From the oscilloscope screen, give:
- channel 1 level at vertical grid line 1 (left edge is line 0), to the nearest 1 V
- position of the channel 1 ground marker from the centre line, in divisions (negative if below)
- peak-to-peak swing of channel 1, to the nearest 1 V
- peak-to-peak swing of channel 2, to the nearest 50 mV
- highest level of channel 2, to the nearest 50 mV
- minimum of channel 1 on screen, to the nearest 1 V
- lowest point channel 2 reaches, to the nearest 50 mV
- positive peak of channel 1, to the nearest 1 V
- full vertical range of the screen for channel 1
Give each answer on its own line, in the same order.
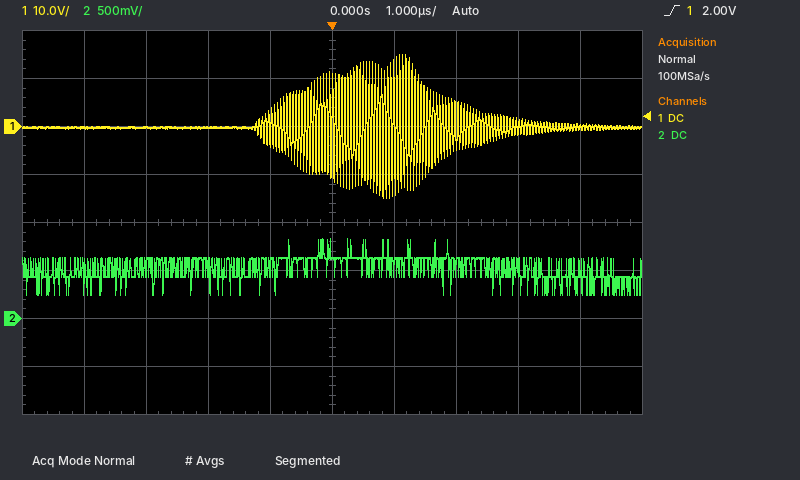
0 V
+2.0 div
30 V
600 mV
850 mV
-15 V
250 mV
15 V
80 V
